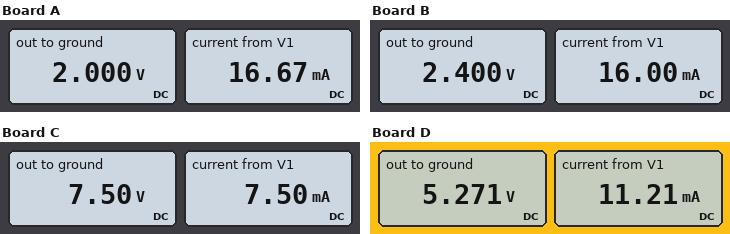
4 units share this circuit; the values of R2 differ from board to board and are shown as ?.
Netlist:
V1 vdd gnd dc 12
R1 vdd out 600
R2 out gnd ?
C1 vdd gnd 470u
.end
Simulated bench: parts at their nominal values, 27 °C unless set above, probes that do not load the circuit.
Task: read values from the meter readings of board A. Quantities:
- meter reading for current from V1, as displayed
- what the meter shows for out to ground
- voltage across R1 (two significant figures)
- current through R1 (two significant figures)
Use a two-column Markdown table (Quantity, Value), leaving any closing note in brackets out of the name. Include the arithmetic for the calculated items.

| Quantity | Value |
|---|---|
| meter reading for current from V1, as displayed | 16.67 mA |
| what the meter shows for out to ground | 2.000 V |
| voltage across R1 | 12 V - 2 V = 10 V |
| current through R1 | (12 V - 2 V) / 600 Ω = 17 mA |
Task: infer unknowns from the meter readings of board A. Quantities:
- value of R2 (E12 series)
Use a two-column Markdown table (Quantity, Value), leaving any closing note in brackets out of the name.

| Quantity | Value |
|---|---|
| value of R2 | 120 Ω |
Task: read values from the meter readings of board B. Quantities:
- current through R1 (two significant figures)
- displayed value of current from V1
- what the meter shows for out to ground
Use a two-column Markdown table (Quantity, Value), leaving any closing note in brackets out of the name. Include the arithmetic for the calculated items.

| Quantity | Value |
|---|---|
| current through R1 | (12 V - 2.4 V) / 600 Ω = 16 mA |
| displayed value of current from V1 | 16.00 mA |
| what the meter shows for out to ground | 2.400 V |
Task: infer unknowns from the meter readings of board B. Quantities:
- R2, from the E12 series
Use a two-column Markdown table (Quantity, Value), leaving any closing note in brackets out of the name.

| Quantity | Value |
|---|---|
| R2, from the E12 series | 150 Ω |
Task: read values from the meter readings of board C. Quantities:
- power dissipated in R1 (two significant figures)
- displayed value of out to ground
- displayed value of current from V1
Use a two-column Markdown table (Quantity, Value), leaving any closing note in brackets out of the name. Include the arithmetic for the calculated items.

| Quantity | Value |
|---|---|
| power dissipated in R1 | (12 V - 7.5 V)^2 / 600 Ω = 34 mW |
| displayed value of out to ground | 7.50 V |
| displayed value of current from V1 | 7.50 mA |
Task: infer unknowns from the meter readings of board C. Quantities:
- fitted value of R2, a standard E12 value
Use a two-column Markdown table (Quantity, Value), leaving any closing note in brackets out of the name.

| Quantity | Value |
|---|---|
| fitted value of R2, a standard E12 value | 1 kΩ |
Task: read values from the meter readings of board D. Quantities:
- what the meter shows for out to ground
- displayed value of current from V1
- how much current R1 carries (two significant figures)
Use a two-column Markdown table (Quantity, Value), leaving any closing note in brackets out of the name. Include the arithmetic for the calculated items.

| Quantity | Value |
|---|---|
| what the meter shows for out to ground | 5.271 V |
| displayed value of current from V1 | 11.21 mA |
| how much current R1 carries | (12 V - 5.271 V) / 600 Ω = 11 mA |
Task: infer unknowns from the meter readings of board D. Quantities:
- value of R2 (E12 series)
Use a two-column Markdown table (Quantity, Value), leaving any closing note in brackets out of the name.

| Quantity | Value |
|---|---|
| value of R2 | 470 Ω |
